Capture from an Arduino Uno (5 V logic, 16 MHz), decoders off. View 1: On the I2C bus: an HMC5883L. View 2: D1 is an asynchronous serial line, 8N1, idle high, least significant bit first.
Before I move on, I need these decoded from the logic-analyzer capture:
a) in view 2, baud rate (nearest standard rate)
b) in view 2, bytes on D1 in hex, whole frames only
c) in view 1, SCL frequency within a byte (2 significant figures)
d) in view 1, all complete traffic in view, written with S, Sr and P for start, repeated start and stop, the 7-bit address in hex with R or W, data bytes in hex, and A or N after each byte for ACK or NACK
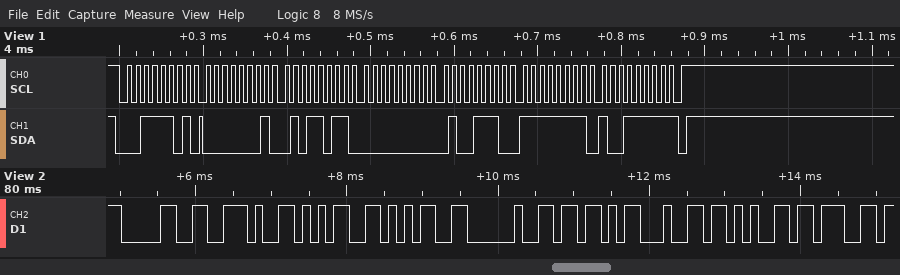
9600 baud
30 2E 35 35 20 5B 64 65 67
100 kHz
S 1ER A 01 A 5B A 00 A 4E A FF A 9F N P
